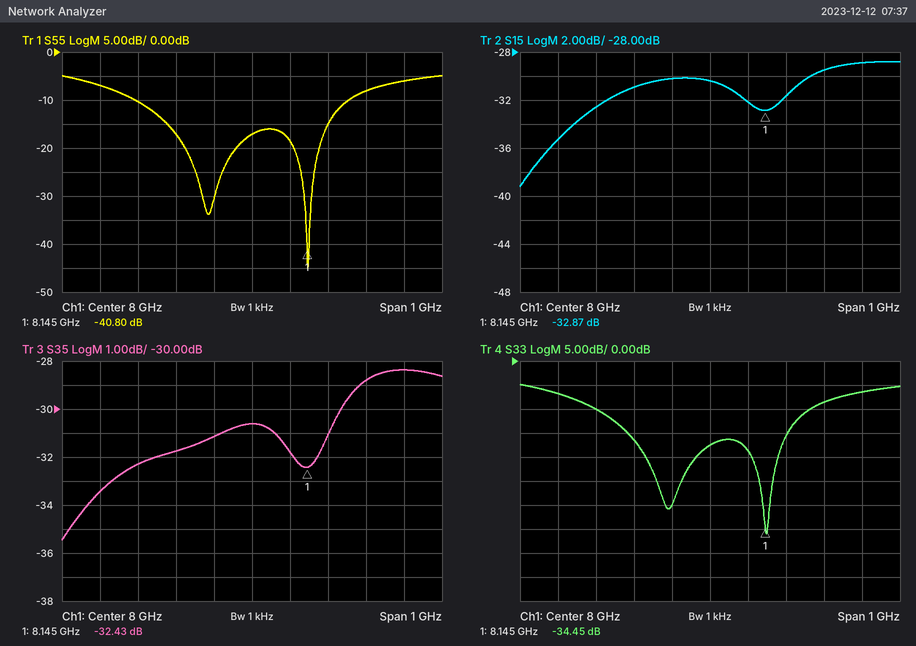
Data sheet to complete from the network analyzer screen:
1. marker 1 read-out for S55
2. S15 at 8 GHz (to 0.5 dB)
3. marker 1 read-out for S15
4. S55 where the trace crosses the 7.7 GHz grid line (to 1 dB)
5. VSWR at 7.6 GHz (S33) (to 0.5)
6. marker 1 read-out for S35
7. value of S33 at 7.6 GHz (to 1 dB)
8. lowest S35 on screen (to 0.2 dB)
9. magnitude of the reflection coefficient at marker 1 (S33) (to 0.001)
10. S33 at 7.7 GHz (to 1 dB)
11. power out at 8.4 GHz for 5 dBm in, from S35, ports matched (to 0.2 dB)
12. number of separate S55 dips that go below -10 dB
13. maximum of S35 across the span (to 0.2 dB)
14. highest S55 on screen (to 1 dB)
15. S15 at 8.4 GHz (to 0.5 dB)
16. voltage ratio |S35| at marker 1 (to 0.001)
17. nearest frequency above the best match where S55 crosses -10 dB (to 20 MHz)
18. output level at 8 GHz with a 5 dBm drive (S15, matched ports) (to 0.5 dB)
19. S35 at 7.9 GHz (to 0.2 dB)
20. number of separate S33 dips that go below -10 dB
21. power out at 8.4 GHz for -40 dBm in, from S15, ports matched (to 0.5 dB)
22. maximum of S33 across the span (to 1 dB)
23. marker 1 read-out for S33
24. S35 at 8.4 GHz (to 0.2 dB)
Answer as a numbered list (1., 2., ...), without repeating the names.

1. -40.80 dB
2. -30.5 dB
3. -32.87 dB
4. -10 dB
5. 2.5
6. -32.43 dB
7. -7 dB
8. -35.4 dB
9. 0.019
10. -10 dB
11. -23.4 dBm
12. 2
13. -28.4 dB
14. -5 dB
15. -29.0 dB
16. 0.024
17. 8.26 GHz
18. -25.5 dBm
19. -31.2 dB
20. 2
21. -69.0 dBm
22. -5 dB
23. -34.45 dB
24. -28.4 dB
